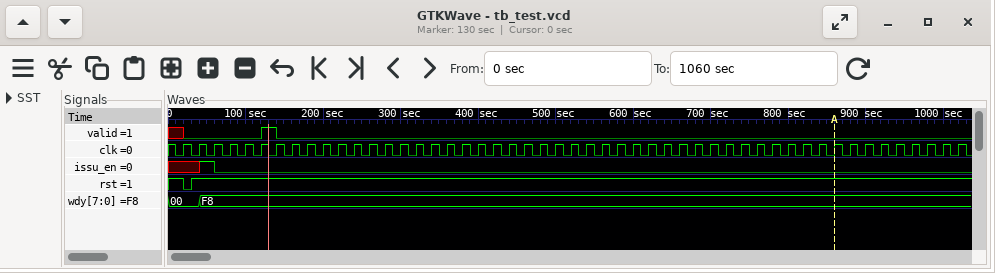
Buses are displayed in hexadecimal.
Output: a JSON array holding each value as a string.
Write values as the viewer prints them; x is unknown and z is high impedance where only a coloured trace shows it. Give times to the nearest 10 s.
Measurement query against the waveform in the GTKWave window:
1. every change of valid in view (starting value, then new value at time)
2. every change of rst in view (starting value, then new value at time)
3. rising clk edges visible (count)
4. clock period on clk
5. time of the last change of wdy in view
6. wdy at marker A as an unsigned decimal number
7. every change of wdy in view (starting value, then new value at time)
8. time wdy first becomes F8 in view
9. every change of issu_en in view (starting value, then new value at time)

["x, 0 at 20 s, 1 at 120 s, 0 at 140 s", "1, 0 at 20 s, 1 at 30 s", "51", "20 s", "40 s", "248", "00, F8 at 40 s", "40 s", "x, 1 at 40 s, 0 at 60 s"]
